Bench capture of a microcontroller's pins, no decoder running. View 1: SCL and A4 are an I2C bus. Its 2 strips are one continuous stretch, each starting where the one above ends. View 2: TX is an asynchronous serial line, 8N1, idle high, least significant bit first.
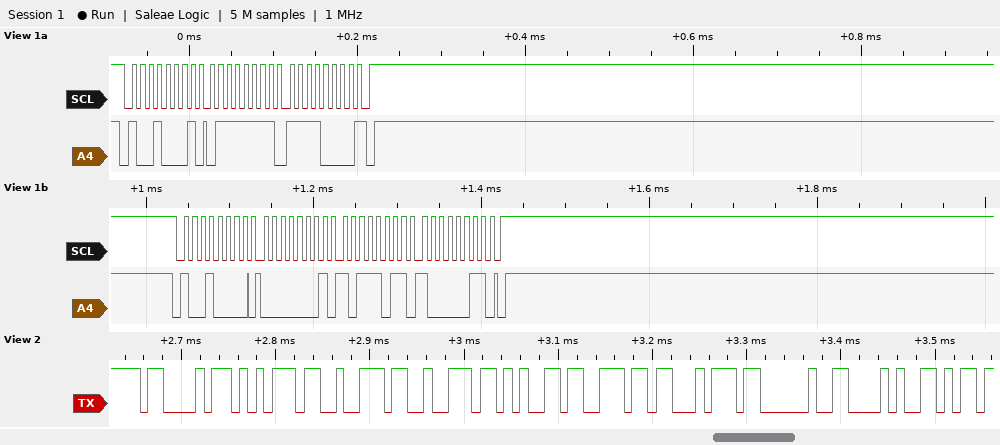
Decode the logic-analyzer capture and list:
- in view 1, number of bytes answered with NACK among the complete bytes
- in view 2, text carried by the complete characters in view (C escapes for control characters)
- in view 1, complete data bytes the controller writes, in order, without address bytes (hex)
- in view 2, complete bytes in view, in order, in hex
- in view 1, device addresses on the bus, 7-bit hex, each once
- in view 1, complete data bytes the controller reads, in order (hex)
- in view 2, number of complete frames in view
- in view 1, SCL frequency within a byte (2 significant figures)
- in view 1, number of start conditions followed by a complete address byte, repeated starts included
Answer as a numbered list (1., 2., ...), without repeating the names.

1. 1
2. "Current ("
3. 01 BB 83
4. 0x43 0x75 0x72 0x72 0x65 0x6E 0x74 0x20 0x28
5. 0x48
6. 7F F0
7. 9
8. 100 kHz
9. 2
